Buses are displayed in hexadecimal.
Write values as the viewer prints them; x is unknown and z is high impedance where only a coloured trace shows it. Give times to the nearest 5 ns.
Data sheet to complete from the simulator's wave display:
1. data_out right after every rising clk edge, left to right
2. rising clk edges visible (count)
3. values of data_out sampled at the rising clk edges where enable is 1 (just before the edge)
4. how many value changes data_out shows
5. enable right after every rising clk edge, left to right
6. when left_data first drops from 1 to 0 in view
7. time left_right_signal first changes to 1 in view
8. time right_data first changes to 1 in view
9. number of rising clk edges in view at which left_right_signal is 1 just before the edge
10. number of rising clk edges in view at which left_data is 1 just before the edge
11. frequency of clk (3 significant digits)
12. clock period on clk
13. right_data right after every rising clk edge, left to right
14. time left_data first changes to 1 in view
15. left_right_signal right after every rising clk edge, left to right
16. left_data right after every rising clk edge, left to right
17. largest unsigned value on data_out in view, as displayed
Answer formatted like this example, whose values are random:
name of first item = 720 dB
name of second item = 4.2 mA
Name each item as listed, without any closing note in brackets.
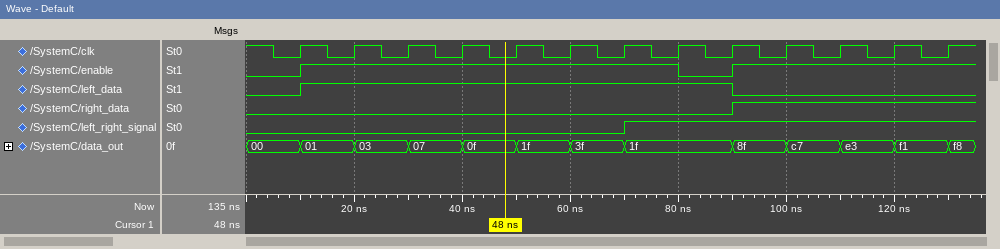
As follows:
data_out right after every rising clk edge, left to right = 01, 03, 07, 0f, 1f, 3f, 1f, 1f, 8f, c7, e3, f1, f8
rising clk edges visible = 13
values of data_out sampled at the rising clk edges where enable is 1 = 01, 03, 07, 0f, 1f, 3f, 1f, 8f, c7, e3, f1
how many value changes data_out shows = 12
enable right after every rising clk edge, left to right = 1 1 1 1 1 1 1 0 1 1 1 1 1
when left_data first drops from 1 to 0 in view = 90 ns
time left_right_signal first changes to 1 in view = 70 ns
time right_data first changes to 1 in view = 90 ns
number of rising clk edges in view at which left_right_signal is 1 just before the edge = 6
number of rising clk edges in view at which left_data is 1 just before the edge = 8
frequency of clk = 100 MHz
clock period on clk = 10 ns
right_data right after every rising clk edge, left to right = 0 0 0 0 0 0 0 0 1 1 1 1 1
time left_data first changes to 1 in view = 10 ns
left_right_signal right after every rising clk edge, left to right = 0 0 0 0 0 0 1 1 1 1 1 1 1
left_data right after every rising clk edge, left to right = 1 1 1 1 1 1 1 1 0 0 0 0 0
largest unsigned value on data_out in view, as displayed = f8
